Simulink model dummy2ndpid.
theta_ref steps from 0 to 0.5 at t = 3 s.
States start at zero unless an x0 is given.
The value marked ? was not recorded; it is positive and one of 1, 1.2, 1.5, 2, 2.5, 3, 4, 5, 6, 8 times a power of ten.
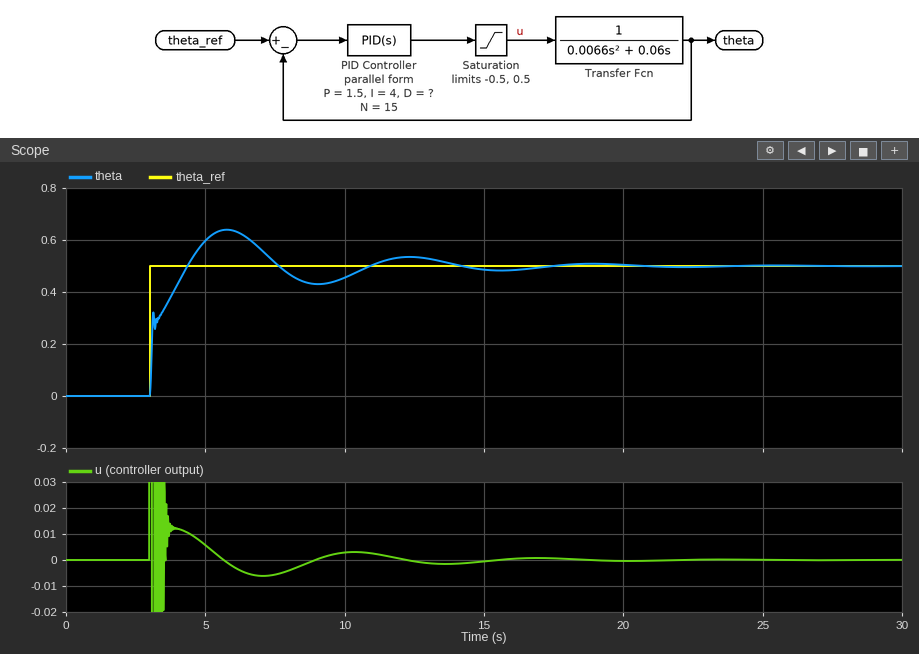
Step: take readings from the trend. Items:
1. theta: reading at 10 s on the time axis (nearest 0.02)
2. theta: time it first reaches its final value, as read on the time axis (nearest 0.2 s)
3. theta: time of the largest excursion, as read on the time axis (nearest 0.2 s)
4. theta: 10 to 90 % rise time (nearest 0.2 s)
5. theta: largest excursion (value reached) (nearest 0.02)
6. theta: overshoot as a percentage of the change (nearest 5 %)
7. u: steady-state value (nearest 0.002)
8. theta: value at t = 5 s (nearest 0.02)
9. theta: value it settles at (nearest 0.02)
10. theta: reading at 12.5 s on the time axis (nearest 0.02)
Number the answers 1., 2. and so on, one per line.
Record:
1. 0.46
2. 4.4 s
3. 5.8 s
4. 1.0 s
5. 0.64
6. 30 %
7. 0.000
8. 0.60
9. 0.50
10. 0.54
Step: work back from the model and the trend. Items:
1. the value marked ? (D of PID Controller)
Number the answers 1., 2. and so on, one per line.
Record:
1. 4
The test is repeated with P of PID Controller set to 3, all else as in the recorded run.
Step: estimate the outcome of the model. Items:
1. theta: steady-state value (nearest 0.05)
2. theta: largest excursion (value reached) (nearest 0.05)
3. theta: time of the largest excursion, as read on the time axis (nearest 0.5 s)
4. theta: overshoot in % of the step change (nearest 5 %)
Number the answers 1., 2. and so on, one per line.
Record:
1. 0.50
2. 0.60
3. 5.5 s
4. 20 %
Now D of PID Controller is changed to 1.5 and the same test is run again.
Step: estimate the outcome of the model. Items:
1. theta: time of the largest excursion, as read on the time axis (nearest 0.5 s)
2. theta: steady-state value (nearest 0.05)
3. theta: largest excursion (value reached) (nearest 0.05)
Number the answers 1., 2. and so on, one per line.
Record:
1. 4.5 s
2. 0.50
3. 0.60
